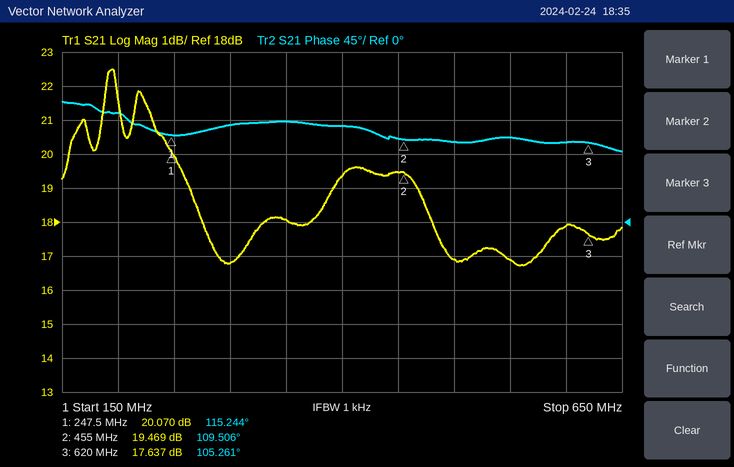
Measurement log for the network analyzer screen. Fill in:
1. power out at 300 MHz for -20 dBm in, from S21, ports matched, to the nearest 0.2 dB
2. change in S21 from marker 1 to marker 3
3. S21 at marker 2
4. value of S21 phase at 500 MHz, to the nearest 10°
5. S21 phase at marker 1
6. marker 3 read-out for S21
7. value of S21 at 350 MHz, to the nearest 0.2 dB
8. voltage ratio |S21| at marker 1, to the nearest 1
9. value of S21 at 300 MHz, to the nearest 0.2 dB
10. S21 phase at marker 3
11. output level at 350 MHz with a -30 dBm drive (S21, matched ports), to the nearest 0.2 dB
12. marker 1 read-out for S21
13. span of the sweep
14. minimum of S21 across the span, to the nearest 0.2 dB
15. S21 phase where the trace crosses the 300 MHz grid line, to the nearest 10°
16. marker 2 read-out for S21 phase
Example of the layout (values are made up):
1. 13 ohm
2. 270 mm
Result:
1. -3.2 dBm
2. -2.433 dB
3. 19.469 dB
4. 110°
5. 115.244°
6. 17.637 dB
7. 18.0 dB
8. 10
9. 16.8 dB
10. 105.261°
11. -12.0 dBm
12. 20.070 dB
13. 500 MHz
14. 16.8 dB
15. 130°
16. 109.506°
